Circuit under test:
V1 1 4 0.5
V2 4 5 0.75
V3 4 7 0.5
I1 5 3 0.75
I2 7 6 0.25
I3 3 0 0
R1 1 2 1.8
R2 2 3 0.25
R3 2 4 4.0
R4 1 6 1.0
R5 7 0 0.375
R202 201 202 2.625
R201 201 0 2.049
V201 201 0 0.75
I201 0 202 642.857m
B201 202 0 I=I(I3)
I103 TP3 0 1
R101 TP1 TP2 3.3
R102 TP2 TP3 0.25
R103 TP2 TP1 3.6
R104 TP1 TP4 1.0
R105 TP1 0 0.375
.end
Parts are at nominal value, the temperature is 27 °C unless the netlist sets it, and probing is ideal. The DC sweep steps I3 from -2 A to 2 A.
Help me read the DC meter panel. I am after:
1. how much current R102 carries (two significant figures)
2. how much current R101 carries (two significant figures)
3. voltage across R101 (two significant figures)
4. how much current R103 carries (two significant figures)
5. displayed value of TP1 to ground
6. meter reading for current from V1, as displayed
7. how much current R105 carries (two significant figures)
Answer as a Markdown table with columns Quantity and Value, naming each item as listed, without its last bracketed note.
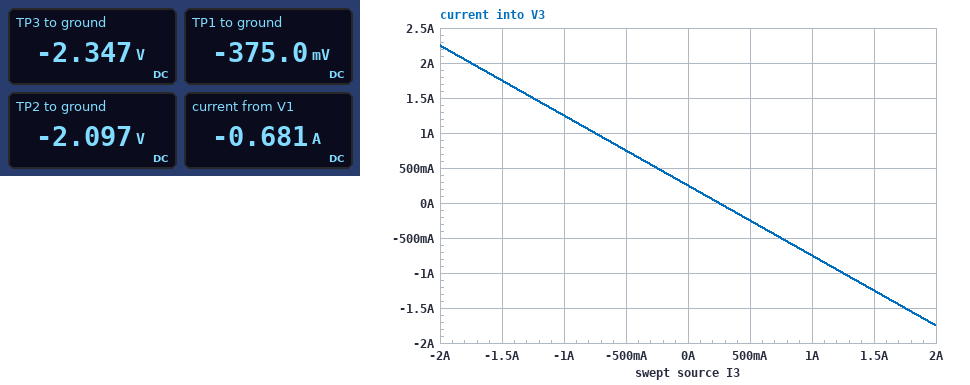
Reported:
| Quantity | Value |
|---|---|
| how much current R102 carries | 1.0 A |
| how much current R101 carries | 520 mA |
| voltage across R101 | 1.7 V |
| how much current R103 carries | 480 mA |
| displayed value of TP1 to ground | -375.0 mV |
| meter reading for current from V1, as displayed | -0.681 A |
| how much current R105 carries | 1.0 A |
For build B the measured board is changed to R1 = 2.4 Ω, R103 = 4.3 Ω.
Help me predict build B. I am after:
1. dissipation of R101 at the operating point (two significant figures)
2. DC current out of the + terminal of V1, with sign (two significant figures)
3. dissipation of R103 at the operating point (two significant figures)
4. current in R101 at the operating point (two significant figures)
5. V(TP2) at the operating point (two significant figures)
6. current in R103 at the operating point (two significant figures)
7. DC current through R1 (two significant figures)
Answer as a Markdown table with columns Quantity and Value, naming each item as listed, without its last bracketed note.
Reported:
| Quantity | Value |
|---|---|
| dissipation of R101 at the operating point | 1.1 W |
| DC current out of the + terminal of V1, with sign | -640 mA |
| dissipation of R103 at the operating point | 810 mW |
| current in R101 at the operating point | 570 mA |
| V(TP2) at the operating point | -2.2 V |
| current in R103 at the operating point | 430 mA |
| DC current through R1 | 390 mA |
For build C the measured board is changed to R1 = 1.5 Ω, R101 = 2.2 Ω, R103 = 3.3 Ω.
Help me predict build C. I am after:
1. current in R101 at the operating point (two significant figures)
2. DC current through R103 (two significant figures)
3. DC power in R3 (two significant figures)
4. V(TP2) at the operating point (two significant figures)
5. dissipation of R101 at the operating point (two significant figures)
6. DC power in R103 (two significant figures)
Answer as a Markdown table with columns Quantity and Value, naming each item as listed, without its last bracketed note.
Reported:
| Quantity | Value |
|---|---|
| current in R101 at the operating point | 600 mA |
| DC current through R103 | 400 mA |
| DC power in R3 | 350 mW |
| V(TP2) at the operating point | -1.7 V |
| dissipation of R101 at the operating point | 790 mW |
| DC power in R103 | 530 mW |
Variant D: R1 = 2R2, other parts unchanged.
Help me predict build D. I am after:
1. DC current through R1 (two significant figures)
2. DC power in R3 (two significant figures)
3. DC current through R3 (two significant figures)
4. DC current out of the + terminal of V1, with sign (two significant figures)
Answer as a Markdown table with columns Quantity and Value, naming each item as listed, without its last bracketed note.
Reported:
| Quantity | Value |
|---|---|
| DC current through R1 | 400 mA |
| DC power in R3 | 480 mW |
| DC current through R3 | 350 mA |
| DC current out of the + terminal of V1, with sign | -650 mA |
